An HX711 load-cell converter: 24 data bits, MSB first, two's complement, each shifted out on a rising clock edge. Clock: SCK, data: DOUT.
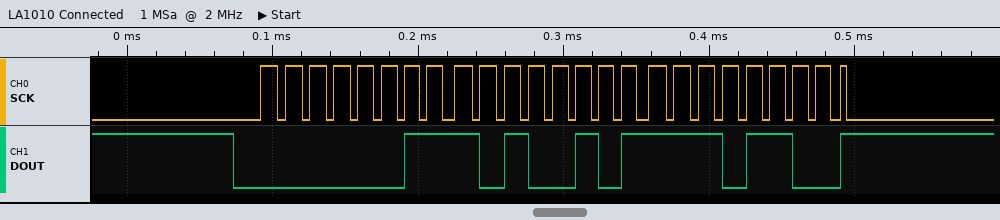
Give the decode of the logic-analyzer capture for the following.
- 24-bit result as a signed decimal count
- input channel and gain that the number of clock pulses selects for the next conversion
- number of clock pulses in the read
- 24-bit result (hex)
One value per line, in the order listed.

239084
channel A, gain 128
25
0x03A5EC
